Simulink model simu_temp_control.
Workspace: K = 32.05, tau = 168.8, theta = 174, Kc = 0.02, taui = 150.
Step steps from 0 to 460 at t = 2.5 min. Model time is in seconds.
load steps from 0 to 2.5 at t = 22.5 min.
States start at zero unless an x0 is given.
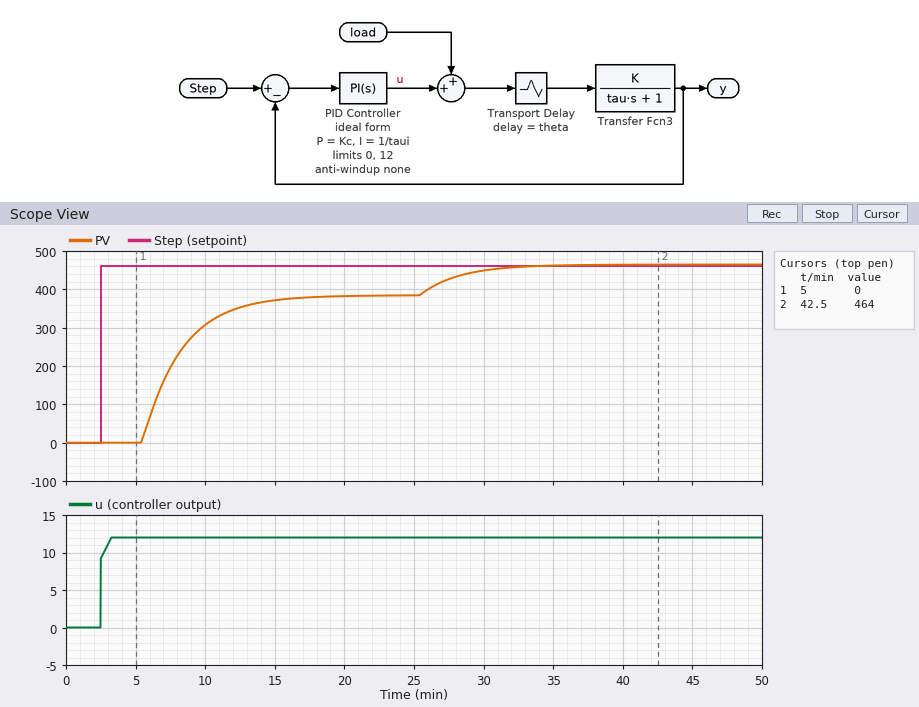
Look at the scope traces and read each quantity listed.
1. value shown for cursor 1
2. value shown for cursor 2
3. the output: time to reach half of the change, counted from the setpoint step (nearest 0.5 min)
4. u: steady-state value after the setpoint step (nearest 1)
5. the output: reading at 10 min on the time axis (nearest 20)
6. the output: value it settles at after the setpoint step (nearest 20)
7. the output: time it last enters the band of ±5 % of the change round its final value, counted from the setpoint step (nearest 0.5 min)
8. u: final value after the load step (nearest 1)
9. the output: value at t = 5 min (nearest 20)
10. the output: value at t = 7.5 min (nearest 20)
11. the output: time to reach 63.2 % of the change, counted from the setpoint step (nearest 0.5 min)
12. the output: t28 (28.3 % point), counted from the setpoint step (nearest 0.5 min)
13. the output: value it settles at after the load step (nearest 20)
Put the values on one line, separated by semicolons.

0; 464; 5.0 min; 12; 300; 380; 11.5 min; 12; 0; 200; 6.0 min; 4.0 min; 460
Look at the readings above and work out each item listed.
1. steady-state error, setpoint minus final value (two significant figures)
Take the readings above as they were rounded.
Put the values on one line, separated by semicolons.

80
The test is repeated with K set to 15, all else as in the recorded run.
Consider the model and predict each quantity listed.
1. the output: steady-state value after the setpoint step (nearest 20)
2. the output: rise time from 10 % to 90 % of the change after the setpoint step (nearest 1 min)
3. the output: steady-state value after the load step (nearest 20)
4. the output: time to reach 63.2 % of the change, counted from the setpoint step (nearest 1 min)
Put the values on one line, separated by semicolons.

180; 6 min; 220; 6 min
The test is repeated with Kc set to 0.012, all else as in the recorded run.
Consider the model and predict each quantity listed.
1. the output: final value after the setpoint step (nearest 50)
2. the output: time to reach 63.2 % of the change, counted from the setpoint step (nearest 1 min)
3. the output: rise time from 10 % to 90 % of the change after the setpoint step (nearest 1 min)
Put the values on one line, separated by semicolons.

400; 7 min; 7 min
